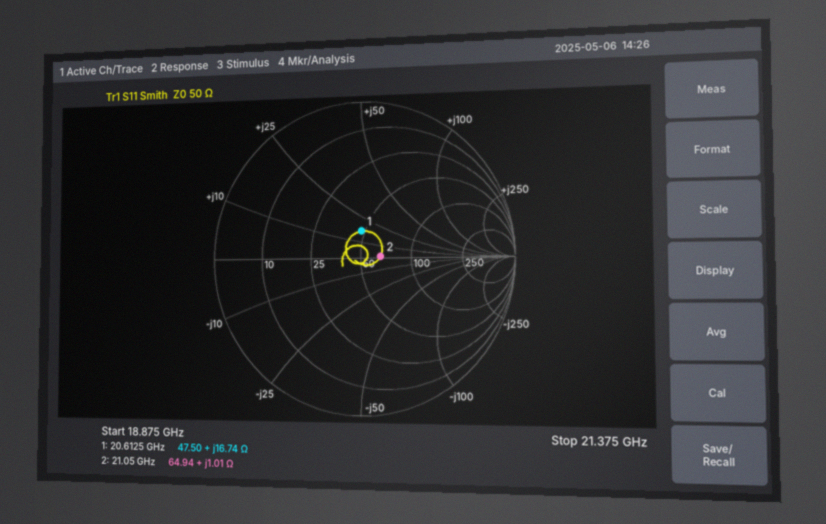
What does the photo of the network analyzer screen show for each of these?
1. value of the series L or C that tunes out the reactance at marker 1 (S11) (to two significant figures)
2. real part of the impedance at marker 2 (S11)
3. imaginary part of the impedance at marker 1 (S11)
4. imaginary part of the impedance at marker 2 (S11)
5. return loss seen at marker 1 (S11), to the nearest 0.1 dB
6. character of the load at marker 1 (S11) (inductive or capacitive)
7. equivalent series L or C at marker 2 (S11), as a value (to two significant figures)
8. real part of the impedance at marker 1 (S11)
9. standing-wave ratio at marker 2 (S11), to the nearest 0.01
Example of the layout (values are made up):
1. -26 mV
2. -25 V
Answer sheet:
1. 460 fF
2. 64.94 Ω
3. +16.74 Ω
4. +1.01 Ω
5. 15.3 dB
6. inductive
7. 7.6 pH
8. 47.50 Ω
9. 1.30
